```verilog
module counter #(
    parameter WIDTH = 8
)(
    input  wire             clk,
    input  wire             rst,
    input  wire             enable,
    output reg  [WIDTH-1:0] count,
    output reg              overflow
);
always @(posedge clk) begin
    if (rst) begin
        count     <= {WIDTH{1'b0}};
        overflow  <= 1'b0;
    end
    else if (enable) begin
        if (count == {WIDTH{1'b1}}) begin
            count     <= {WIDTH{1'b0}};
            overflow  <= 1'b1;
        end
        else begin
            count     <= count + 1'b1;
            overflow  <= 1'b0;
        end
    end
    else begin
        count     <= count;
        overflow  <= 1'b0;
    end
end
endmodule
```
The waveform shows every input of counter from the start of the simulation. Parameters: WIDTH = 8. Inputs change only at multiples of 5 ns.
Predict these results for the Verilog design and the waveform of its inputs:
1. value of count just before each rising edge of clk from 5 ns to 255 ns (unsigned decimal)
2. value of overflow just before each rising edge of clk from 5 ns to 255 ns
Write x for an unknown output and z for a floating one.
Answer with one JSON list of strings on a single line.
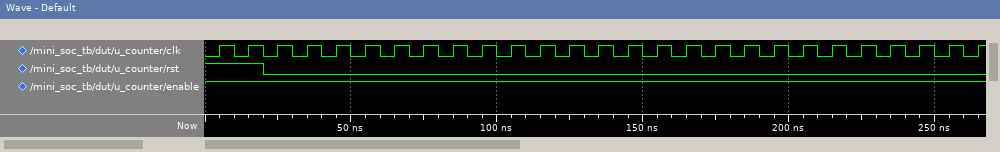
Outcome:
["x, 0, 0, 1, 2, 3, 4, 5, 6, 7, 8, 9, 10, 11, 12, 13, 14, 15, 16, 17, 18, 19, 20, 21, 22, 23", "x 0 0 0 0 0 0 0 0 0 0 0 0 0 0 0 0 0 0 0 0 0 0 0 0 0"]
